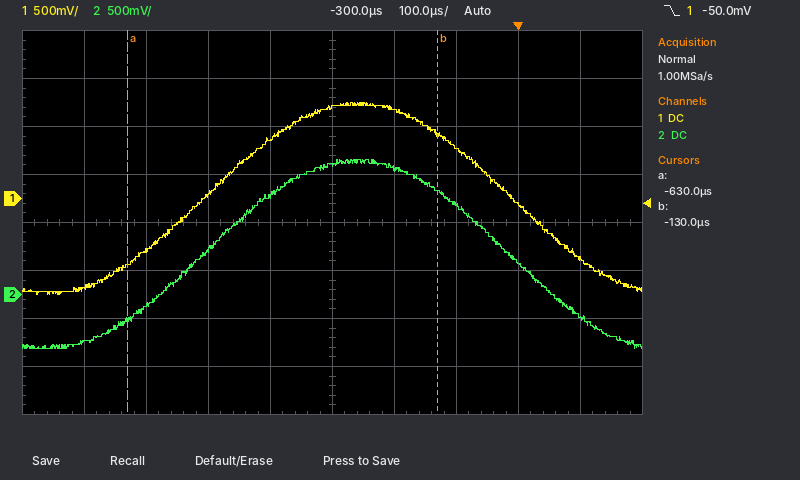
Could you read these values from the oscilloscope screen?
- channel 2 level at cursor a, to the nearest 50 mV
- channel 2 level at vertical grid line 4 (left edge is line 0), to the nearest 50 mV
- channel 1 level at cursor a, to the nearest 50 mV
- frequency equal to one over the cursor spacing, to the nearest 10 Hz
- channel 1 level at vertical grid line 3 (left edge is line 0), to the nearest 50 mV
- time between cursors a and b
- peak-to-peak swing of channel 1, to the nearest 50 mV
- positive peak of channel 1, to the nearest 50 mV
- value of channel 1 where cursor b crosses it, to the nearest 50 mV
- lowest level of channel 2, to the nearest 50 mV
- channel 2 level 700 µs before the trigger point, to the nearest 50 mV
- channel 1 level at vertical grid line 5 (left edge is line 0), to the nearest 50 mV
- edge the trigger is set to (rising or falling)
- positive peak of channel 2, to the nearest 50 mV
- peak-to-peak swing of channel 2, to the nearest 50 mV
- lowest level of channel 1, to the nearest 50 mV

-250 mV
1.05 V
-700 mV
2.00 kHz
50 mV
500 µs
2.00 V
1.00 V
700 mV
-550 mV
-500 mV
950 mV
falling
1.40 V
1.95 V
-1.00 V
